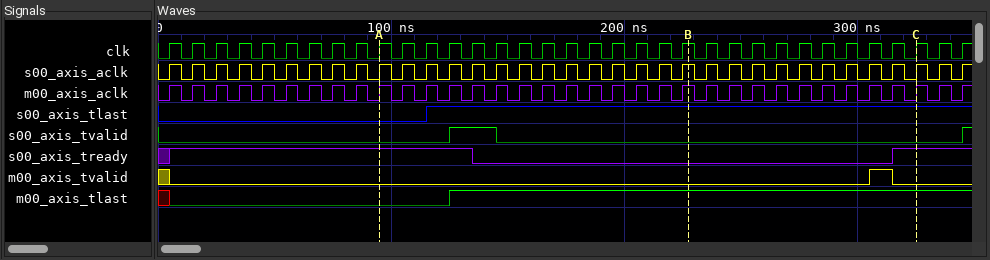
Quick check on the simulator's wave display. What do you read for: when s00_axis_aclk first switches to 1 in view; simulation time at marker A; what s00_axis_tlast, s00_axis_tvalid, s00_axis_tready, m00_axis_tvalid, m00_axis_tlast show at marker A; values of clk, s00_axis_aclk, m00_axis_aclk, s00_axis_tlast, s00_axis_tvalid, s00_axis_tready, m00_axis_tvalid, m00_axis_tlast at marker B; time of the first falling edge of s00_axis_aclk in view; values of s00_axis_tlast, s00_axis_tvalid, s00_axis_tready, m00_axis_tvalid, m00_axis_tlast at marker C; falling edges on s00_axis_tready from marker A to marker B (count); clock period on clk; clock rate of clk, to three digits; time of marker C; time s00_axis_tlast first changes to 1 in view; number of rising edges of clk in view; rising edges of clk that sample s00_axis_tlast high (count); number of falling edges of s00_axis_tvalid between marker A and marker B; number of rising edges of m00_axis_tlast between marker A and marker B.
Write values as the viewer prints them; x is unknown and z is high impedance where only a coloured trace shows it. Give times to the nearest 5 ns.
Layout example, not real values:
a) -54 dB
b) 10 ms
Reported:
a) 5 ns
b) 95 ns
c) s00_axis_tlast=0, s00_axis_tvalid=0, s00_axis_tready=1, m00_axis_tvalid=0, m00_axis_tlast=0
d) clk=1, s00_axis_aclk=1, m00_axis_aclk=1, s00_axis_tlast=1, s00_axis_tvalid=0, s00_axis_tready=0, m00_axis_tvalid=0, m00_axis_tlast=1
e) 10 ns
f) s00_axis_tlast=1, s00_axis_tvalid=0, s00_axis_tready=1, m00_axis_tvalid=0, m00_axis_tlast=1
g) 1
h) 10 ns
i) 100 MHz
j) 325 ns
k) 115 ns
l) 35
m) 23
n) 1
o) 1
